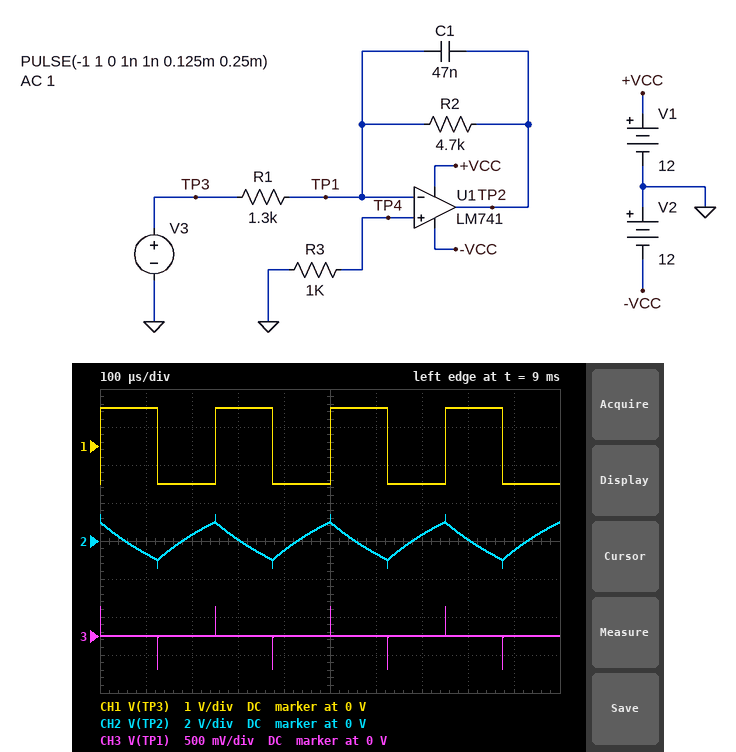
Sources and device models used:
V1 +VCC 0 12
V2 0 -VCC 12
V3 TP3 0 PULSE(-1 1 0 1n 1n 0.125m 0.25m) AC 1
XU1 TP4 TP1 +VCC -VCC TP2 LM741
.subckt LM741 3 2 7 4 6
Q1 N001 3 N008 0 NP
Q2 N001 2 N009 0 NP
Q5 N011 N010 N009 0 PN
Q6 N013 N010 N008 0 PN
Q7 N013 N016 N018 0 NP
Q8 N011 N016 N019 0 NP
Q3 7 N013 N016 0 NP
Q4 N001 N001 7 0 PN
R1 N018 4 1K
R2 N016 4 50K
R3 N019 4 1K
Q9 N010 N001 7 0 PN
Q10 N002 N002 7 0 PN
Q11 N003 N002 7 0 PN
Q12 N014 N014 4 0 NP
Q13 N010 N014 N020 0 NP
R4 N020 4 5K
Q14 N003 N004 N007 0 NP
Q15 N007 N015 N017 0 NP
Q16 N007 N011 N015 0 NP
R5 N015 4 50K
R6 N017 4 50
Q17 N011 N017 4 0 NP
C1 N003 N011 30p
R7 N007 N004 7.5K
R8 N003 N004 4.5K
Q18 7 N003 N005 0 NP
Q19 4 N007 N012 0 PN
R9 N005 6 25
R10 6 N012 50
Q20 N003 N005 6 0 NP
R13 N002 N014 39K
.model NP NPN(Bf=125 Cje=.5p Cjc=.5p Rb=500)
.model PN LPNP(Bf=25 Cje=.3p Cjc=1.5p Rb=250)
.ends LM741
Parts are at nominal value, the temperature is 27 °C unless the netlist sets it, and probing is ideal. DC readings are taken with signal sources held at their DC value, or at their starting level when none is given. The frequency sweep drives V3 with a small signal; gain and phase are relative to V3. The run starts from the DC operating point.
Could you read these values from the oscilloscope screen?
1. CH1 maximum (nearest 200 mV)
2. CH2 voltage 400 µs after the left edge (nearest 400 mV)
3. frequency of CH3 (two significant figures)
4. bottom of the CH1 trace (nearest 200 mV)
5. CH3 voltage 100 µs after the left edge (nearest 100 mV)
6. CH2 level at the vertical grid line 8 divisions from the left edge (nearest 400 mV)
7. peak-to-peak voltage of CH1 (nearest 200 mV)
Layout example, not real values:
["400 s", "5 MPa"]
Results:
["1.0 V", "-400 mV", "4.0 kHz", "-1.0 V", "0 V", "0 V", "2.0 V"]
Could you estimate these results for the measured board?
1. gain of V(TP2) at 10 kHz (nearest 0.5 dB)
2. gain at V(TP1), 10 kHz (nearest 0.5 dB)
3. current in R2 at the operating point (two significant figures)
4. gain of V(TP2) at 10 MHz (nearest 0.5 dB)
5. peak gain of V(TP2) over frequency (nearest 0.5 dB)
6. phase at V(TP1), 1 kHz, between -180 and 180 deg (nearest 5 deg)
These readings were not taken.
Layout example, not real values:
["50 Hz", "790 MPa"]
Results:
["-11.5 dB", "-51.0 dB", "770 µA", "-26.5 dB", "11.0 dB", "35 deg"]
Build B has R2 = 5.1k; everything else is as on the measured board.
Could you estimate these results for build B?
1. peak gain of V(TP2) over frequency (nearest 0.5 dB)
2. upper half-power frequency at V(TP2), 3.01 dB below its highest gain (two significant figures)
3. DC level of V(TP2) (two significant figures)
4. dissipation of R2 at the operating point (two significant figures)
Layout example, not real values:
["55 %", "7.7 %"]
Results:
["12.0 dB", "660 Hz", "3.9 V", "3.0 mW"]
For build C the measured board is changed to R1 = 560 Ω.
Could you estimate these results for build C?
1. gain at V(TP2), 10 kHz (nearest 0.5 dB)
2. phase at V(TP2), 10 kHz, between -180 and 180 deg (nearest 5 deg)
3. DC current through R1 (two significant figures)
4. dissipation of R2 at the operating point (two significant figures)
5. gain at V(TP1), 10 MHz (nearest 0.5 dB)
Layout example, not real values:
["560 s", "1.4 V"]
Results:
["-4.5 dB", "95 deg", "1.8 mA", "15 mW", "-22.5 dB"]
